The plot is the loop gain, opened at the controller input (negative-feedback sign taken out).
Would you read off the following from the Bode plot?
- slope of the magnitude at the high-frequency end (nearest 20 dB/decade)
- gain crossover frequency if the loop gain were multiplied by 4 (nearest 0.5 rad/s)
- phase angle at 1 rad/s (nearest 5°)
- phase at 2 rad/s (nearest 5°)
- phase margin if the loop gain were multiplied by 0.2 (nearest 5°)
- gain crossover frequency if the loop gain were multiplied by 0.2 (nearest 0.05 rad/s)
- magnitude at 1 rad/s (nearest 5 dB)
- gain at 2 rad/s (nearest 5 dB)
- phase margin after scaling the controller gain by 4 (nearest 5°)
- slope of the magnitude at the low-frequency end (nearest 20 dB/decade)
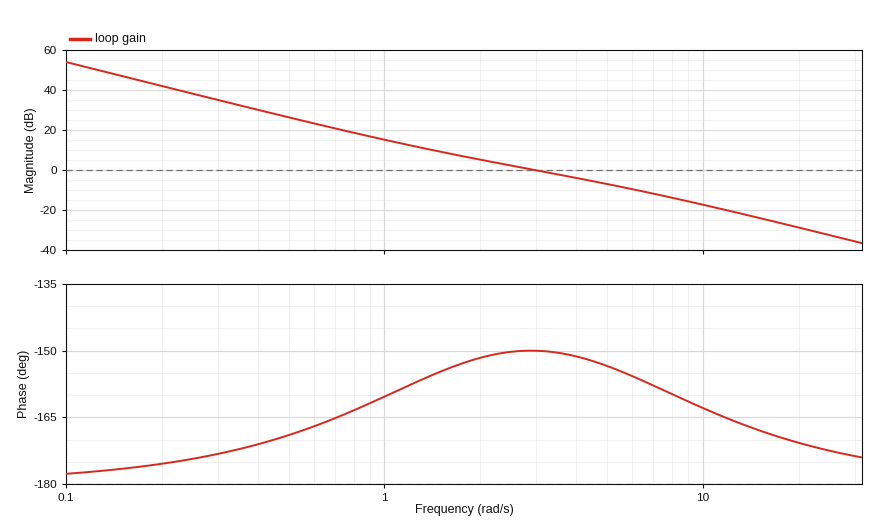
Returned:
-40 dB/decade
7.0 rad/s
-160°
-150°
20°
1.10 rad/s
15 dB
5 dB
20°
-40 dB/decade
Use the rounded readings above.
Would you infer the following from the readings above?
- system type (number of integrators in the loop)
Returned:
2
